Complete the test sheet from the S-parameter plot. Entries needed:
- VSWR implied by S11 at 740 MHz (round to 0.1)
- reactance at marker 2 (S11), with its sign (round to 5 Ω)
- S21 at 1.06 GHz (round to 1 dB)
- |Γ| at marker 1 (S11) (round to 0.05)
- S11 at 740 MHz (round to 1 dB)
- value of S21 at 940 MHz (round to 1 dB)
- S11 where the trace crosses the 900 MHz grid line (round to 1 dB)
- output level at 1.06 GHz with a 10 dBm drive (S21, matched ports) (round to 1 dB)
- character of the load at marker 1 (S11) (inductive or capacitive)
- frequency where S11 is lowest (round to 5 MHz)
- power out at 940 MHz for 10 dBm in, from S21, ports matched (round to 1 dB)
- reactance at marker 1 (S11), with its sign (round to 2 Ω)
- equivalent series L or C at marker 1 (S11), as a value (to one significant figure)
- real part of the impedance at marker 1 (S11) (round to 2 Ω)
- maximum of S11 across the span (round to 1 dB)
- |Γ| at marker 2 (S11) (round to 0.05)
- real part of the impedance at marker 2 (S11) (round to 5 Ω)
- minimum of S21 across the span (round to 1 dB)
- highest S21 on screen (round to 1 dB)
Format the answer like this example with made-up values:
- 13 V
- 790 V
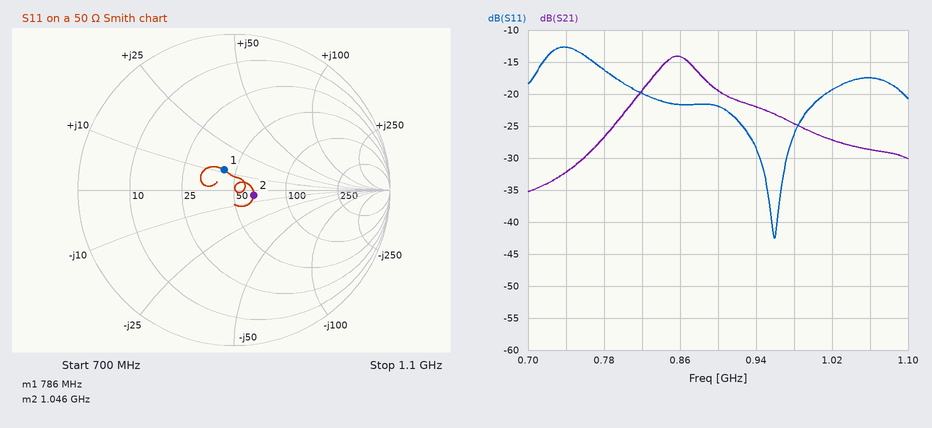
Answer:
- 1.6
- -5 Ω
- -29 dB
- 0.15
- -13 dB
- -22 dB
- -22 dB
- -19 dBm
- inductive
- 960 MHz
- -12 dBm
- +12 Ω
- 2 nH
- 42 Ω
- -13 dB
- 0.15
- 65 Ω
- -35 dB
- -14 dB
